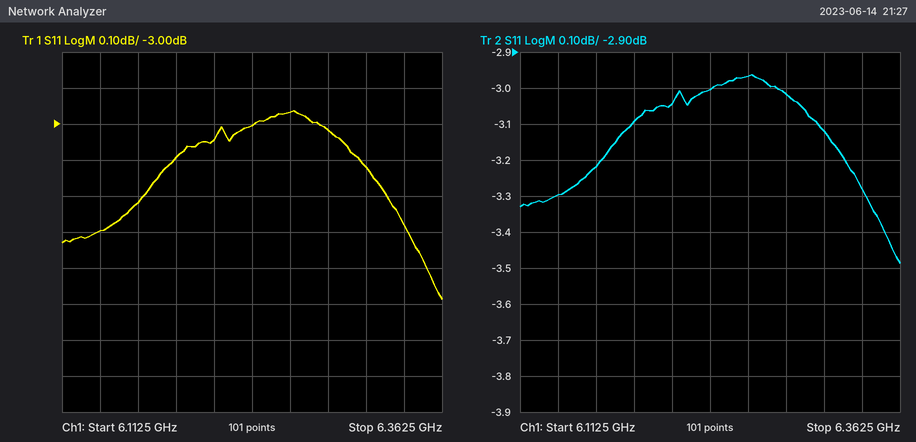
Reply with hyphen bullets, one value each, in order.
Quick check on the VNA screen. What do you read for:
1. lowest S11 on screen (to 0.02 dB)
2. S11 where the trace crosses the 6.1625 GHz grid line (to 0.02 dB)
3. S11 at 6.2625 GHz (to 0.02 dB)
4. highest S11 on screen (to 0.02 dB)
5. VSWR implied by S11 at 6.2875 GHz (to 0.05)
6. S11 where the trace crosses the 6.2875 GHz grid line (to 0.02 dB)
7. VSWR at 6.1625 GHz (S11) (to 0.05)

- -3.48 dB
- -3.22 dB
- -2.96 dB
- -2.96 dB
- 5.80
- -3.02 dB
- 5.45
